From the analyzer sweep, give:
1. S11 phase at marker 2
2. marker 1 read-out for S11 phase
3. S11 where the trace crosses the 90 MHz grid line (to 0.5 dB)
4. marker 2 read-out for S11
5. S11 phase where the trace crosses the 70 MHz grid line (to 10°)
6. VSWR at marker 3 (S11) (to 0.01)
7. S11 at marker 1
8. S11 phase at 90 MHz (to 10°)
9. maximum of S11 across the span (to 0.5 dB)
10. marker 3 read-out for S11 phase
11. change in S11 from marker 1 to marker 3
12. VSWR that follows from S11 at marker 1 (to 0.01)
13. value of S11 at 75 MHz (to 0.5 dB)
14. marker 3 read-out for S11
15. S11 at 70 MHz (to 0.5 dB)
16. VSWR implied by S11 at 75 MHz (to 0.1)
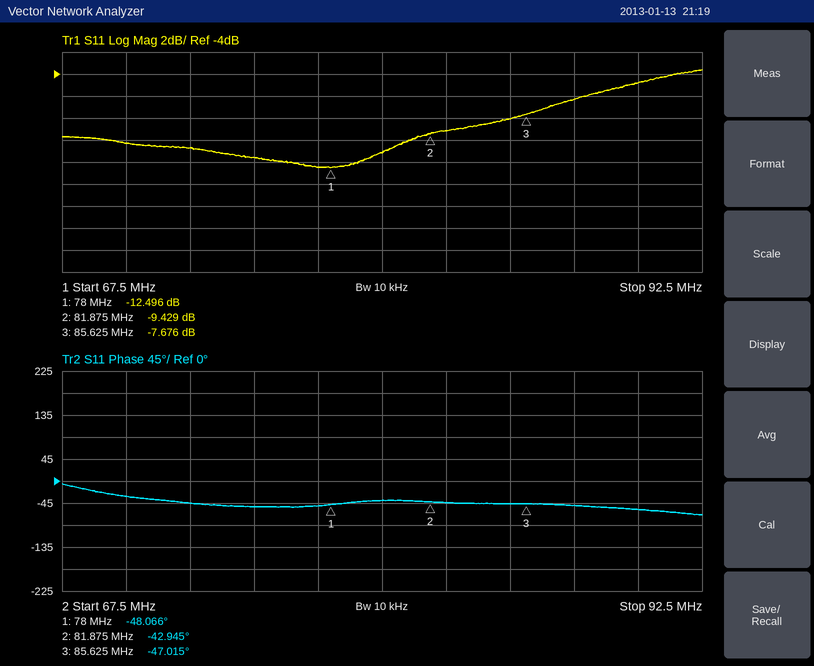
-42.945°
-48.066°
-5.0 dB
-9.429 dB
-30°
2.41
-12.496 dB
-60°
-3.5 dB
-47.015°
4.820 dB
1.62
-11.5 dB
-7.676 dB
-10.5 dB
1.7
